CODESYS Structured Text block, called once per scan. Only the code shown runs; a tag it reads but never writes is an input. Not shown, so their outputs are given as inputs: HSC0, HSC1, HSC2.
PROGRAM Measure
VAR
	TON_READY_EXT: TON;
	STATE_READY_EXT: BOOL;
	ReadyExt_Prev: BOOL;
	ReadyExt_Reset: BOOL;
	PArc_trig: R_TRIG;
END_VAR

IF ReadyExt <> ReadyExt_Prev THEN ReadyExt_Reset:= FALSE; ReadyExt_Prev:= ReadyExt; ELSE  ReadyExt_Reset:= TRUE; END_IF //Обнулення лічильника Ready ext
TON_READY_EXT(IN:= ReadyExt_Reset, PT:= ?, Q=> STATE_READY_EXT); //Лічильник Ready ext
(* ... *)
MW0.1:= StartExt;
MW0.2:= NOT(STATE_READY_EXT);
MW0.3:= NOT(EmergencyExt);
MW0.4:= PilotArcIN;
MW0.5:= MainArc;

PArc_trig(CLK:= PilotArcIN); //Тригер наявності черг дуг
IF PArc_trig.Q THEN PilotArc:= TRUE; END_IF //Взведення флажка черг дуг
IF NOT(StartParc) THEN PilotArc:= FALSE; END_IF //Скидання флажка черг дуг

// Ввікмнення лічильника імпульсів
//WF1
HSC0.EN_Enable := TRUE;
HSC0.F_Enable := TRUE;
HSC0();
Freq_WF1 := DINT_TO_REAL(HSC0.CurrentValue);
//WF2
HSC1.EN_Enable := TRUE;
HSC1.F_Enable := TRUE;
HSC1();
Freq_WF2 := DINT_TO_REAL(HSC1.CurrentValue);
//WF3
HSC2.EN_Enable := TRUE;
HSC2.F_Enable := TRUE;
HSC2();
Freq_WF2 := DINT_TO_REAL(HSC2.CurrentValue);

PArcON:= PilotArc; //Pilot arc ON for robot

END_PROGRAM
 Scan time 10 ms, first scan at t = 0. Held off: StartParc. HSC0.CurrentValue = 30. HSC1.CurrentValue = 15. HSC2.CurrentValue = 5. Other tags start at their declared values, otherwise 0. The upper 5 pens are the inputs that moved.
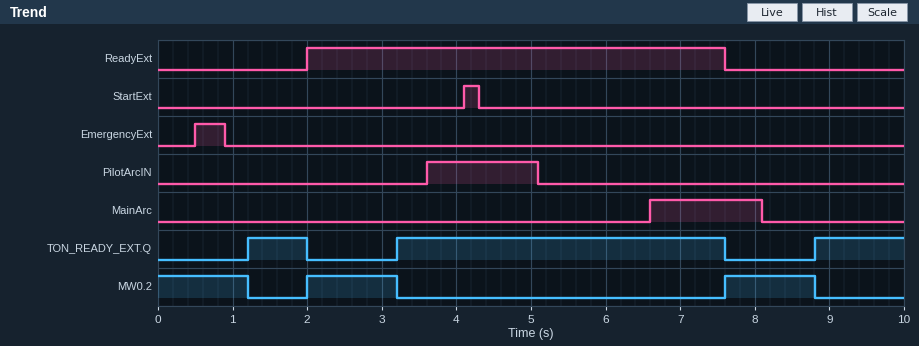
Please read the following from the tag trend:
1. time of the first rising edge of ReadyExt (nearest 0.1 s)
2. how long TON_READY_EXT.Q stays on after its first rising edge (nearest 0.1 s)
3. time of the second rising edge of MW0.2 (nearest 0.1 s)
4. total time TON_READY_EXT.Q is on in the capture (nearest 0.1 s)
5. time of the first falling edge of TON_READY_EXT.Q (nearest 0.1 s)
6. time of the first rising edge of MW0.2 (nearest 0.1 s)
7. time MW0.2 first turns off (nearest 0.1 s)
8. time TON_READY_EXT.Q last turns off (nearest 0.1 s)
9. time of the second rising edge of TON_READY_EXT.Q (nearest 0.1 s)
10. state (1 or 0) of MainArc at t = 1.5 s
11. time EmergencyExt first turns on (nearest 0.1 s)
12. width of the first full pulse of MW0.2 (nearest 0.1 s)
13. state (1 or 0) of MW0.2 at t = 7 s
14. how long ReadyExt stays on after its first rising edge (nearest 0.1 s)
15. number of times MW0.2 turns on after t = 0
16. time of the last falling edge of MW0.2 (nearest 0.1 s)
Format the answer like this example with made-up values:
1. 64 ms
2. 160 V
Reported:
1. 2.0 s
2. 0.8 s
3. 7.6 s
4. 6.4 s
5. 2.0 s
6. 2.0 s
7. 1.2 s
8. 7.6 s
9. 3.2 s
10. 0
11. 0.5 s
12. 1.2 s
13. 0
14. 5.6 s
15. 2
16. 8.8 s
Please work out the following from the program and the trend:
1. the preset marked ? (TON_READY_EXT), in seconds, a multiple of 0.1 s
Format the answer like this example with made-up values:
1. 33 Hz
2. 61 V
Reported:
1. 1.2 s
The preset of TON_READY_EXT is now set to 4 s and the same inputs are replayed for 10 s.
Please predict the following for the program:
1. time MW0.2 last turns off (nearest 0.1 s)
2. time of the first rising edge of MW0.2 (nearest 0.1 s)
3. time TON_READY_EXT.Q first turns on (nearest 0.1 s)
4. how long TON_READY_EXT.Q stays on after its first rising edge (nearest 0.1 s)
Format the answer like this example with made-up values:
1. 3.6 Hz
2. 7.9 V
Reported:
1. 6.0 s
2. 7.6 s
3. 6.0 s
4. 1.6 s
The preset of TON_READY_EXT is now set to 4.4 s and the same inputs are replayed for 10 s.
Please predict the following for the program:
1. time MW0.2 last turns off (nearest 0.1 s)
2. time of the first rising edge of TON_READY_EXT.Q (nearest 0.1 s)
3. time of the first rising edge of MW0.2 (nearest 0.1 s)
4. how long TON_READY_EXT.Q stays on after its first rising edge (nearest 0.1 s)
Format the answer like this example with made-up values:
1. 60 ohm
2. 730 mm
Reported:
1. 6.4 s
2. 6.4 s
3. 7.6 s
4. 1.2 s
